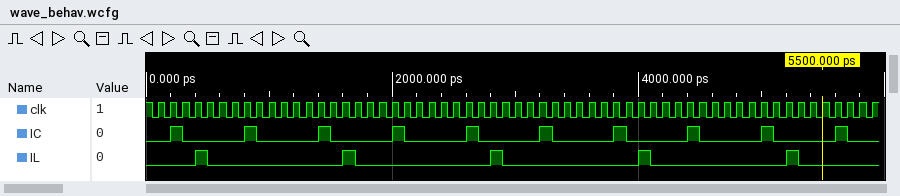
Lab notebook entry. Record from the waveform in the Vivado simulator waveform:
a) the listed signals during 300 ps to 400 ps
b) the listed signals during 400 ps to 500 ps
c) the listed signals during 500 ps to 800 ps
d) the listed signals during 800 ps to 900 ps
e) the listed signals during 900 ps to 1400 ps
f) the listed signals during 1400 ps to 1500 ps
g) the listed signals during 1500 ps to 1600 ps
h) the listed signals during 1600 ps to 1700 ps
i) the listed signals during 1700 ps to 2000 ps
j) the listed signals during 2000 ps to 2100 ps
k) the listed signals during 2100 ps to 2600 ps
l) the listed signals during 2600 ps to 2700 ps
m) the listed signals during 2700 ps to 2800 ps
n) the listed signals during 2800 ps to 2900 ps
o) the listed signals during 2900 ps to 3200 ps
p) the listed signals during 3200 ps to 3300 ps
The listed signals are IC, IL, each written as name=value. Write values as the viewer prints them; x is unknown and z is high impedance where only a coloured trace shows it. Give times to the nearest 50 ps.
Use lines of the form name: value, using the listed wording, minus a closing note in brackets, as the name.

the listed signals during 300 ps to 400 ps: IC=0, IL=0
the listed signals during 400 ps to 500 ps: IC=0, IL=1
the listed signals during 500 ps to 800 ps: IC=0, IL=0
the listed signals during 800 ps to 900 ps: IC=1, IL=0
the listed signals during 900 ps to 1400 ps: IC=0, IL=0
the listed signals during 1400 ps to 1500 ps: IC=1, IL=0
the listed signals during 1500 ps to 1600 ps: IC=0, IL=0
the listed signals during 1600 ps to 1700 ps: IC=0, IL=1
the listed signals during 1700 ps to 2000 ps: IC=0, IL=0
the listed signals during 2000 ps to 2100 ps: IC=1, IL=0
the listed signals during 2100 ps to 2600 ps: IC=0, IL=0
the listed signals during 2600 ps to 2700 ps: IC=1, IL=0
the listed signals during 2700 ps to 2800 ps: IC=0, IL=0
the listed signals during 2800 ps to 2900 ps: IC=0, IL=1
the listed signals during 2900 ps to 3200 ps: IC=0, IL=0
the listed signals during 3200 ps to 3300 ps: IC=1, IL=0
